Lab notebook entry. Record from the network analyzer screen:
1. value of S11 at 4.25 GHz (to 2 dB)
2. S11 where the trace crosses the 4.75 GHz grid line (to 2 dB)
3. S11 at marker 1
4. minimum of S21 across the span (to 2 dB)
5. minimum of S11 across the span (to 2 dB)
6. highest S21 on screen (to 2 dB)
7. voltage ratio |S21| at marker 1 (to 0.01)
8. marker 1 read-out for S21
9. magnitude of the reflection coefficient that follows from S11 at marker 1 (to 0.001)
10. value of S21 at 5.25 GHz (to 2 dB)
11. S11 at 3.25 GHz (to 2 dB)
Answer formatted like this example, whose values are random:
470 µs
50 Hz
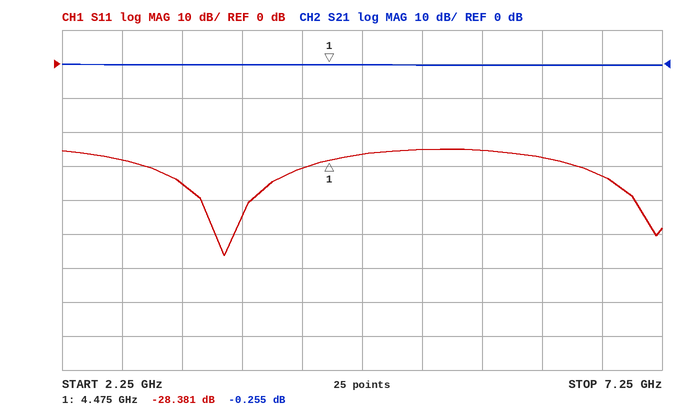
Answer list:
-30 dB
-26 dB
-28.381 dB
0 dB
-56 dB
0 dB
0.97
-0.255 dB
0.038
0 dB
-36 dB
